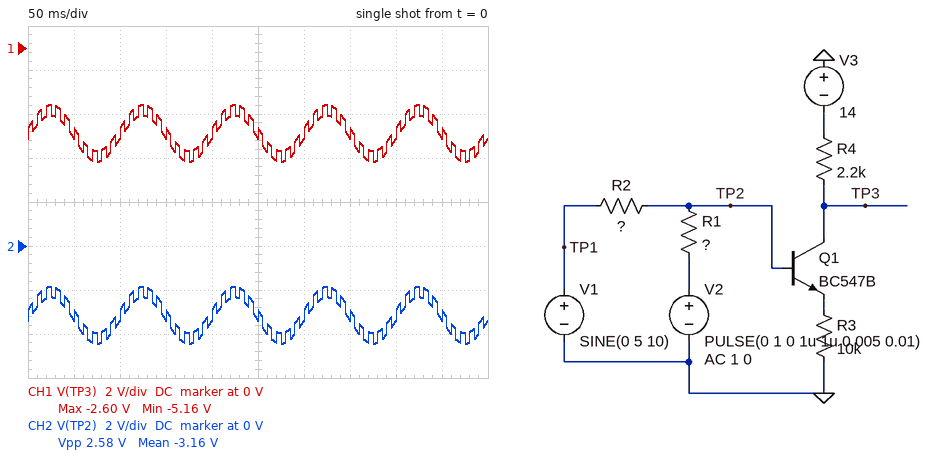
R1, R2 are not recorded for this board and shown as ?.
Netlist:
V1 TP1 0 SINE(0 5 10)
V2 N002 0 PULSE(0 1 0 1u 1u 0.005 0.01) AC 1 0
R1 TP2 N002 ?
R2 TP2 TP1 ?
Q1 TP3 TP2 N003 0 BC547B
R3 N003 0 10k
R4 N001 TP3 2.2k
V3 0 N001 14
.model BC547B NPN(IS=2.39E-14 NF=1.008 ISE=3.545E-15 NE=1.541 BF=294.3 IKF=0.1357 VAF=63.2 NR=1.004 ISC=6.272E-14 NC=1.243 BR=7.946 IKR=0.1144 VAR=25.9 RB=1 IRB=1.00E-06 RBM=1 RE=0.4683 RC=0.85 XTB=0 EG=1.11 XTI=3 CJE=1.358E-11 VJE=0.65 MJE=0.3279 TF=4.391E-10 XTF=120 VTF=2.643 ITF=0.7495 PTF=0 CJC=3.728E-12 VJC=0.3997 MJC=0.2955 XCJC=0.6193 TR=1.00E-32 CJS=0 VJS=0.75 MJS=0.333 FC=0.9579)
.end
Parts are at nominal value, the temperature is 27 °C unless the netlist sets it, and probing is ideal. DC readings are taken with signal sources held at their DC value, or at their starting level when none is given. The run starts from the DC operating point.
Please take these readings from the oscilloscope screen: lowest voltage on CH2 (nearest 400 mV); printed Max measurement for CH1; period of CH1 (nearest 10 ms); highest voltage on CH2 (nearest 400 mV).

-4.4 V
-2.60 V
100 ms
-2.0 V
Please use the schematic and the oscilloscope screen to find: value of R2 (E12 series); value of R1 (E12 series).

2.7 kΩ
1.2 kΩ
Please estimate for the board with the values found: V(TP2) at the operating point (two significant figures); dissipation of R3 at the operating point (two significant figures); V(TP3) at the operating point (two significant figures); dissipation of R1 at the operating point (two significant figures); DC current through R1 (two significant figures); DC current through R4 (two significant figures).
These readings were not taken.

-3.4 V
1.7 mW
-4.1 V
9.6 mW
2.8 mA
4.5 mA
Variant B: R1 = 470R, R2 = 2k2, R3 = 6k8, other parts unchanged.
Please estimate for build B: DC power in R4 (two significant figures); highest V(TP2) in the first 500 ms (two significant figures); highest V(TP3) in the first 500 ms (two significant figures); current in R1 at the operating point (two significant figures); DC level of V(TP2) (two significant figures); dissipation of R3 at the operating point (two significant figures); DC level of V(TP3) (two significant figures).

59 mW
-480 mV
-1.2 V
4.0 mA
-1.9 V
990 µW
-2.6 V
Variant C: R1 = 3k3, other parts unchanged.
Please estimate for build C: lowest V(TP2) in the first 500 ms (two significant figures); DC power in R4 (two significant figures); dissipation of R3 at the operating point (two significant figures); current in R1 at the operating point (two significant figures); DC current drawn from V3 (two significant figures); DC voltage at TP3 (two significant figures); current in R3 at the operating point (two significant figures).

-6.4 V
32 mW
3.1 mW
1.5 mA
3.8 mA
-5.6 V
560 µA
